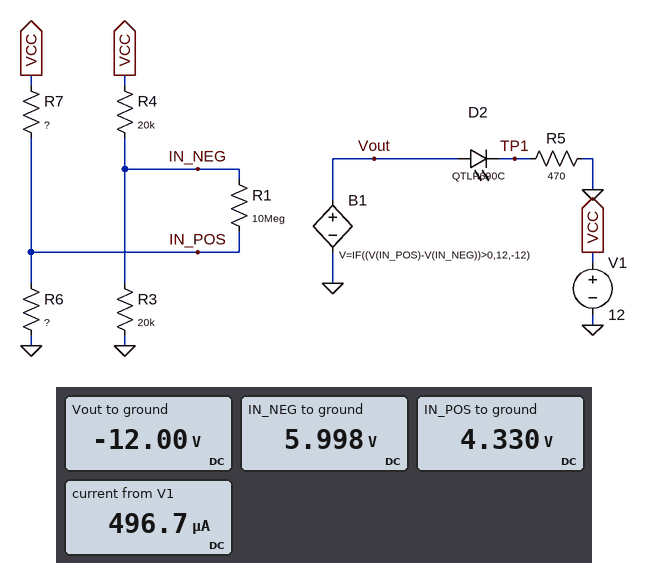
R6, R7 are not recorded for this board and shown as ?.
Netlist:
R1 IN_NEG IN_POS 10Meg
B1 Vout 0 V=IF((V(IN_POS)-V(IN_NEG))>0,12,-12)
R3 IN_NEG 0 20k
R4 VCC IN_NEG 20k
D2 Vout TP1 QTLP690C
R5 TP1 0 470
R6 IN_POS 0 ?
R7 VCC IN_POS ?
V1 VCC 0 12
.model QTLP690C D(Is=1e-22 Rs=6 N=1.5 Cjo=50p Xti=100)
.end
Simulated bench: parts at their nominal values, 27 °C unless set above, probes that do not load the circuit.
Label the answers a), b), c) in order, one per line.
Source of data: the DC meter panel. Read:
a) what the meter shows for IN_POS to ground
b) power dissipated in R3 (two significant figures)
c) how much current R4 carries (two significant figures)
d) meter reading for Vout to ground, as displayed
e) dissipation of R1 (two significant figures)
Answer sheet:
a) 4.330 V
b) 1.8 mW
c) 300 µA
d) -12.00 V
e) 280 nW
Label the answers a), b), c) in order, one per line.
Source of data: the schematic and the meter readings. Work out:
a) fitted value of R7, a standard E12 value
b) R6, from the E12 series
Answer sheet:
a) 39 kΩ
b) 22 kΩ
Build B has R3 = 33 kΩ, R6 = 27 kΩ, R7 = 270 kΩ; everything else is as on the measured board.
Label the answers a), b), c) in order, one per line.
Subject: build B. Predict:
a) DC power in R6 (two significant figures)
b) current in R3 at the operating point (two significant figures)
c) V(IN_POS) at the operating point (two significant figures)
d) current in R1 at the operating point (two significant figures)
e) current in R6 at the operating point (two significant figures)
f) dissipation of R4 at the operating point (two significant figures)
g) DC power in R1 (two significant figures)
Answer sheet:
a) 45 µW
b) 230 µA
c) 1.1 V
d) 640 nA
e) 41 µA
f) 1.0 mW
g) 4.0 µW
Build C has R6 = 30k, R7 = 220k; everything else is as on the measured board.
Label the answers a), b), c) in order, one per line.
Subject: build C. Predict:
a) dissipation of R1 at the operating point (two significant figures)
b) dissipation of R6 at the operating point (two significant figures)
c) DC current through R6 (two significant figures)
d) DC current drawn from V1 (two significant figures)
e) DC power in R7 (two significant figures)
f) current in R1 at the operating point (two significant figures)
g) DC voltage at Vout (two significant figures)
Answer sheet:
a) 2.1 µW
b) 70 µW
c) 48 µA
d) 350 µA
e) 510 µW
f) 450 nA
g) -12 V
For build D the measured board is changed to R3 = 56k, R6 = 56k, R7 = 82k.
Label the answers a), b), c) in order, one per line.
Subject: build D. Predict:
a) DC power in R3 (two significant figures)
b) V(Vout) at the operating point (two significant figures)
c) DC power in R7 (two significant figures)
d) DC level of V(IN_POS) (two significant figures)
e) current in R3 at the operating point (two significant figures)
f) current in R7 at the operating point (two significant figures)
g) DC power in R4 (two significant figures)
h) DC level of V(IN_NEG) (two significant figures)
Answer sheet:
a) 1.4 mW
b) -12 V
c) 620 µW
d) 4.9 V
e) 160 µA
f) 87 µA
g) 500 µW
h) 8.8 V
